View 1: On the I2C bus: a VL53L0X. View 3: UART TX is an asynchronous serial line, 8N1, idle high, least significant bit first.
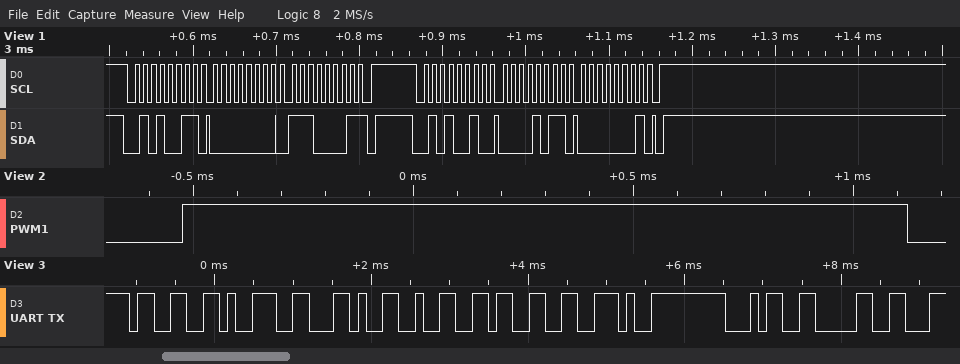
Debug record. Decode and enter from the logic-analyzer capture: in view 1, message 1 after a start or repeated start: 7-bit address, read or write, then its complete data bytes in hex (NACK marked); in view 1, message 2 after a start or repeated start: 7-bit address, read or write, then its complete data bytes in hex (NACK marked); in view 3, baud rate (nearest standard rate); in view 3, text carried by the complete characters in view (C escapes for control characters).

0x29 read: 00 E1 NACK
0x29 write: 0B 01
9600 baud
"39,23.40"
